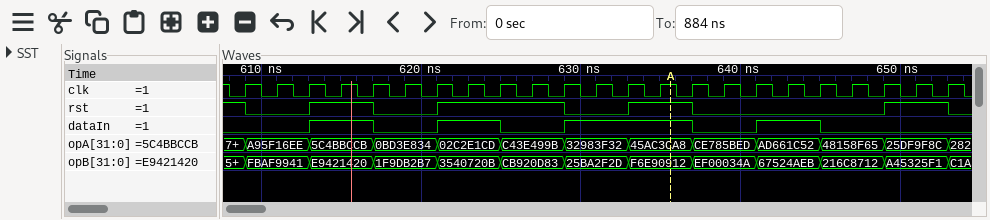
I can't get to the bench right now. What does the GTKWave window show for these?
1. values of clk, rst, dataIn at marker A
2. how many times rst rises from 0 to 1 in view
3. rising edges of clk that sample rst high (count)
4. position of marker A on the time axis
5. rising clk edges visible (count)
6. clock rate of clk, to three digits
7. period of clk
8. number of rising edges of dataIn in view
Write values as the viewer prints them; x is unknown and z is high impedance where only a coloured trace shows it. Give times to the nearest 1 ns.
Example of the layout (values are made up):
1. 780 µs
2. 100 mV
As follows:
1. clk=1, rst=1, dataIn=1
2. 4
3. 11
4. 636 ns
5. 23
6. 500 MHz
7. 2 ns
8. 4
